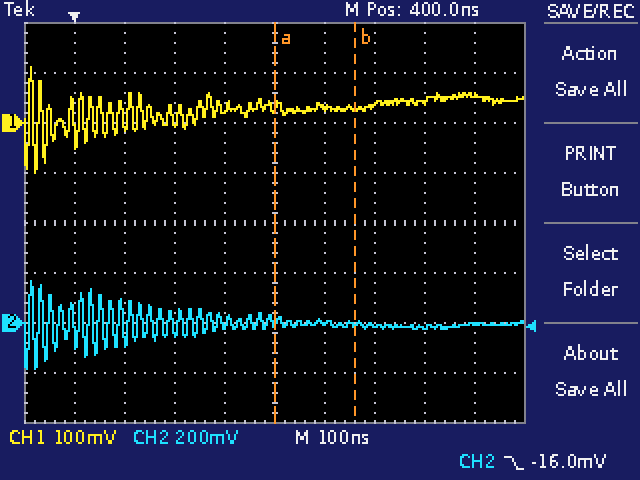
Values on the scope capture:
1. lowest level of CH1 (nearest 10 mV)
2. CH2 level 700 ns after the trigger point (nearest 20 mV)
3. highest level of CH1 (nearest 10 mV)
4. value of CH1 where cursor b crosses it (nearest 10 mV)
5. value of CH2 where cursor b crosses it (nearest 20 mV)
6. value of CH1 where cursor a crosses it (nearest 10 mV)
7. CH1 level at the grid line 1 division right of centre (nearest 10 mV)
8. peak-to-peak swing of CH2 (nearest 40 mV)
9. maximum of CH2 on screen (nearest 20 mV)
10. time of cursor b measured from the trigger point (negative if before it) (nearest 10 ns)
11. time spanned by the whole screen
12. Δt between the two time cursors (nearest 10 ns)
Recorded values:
-100 mV
-20 mV
110 mV
30 mV
0 mV
30 mV
30 mV
360 mV
160 mV
+560 ns
1 µs
160 ns
